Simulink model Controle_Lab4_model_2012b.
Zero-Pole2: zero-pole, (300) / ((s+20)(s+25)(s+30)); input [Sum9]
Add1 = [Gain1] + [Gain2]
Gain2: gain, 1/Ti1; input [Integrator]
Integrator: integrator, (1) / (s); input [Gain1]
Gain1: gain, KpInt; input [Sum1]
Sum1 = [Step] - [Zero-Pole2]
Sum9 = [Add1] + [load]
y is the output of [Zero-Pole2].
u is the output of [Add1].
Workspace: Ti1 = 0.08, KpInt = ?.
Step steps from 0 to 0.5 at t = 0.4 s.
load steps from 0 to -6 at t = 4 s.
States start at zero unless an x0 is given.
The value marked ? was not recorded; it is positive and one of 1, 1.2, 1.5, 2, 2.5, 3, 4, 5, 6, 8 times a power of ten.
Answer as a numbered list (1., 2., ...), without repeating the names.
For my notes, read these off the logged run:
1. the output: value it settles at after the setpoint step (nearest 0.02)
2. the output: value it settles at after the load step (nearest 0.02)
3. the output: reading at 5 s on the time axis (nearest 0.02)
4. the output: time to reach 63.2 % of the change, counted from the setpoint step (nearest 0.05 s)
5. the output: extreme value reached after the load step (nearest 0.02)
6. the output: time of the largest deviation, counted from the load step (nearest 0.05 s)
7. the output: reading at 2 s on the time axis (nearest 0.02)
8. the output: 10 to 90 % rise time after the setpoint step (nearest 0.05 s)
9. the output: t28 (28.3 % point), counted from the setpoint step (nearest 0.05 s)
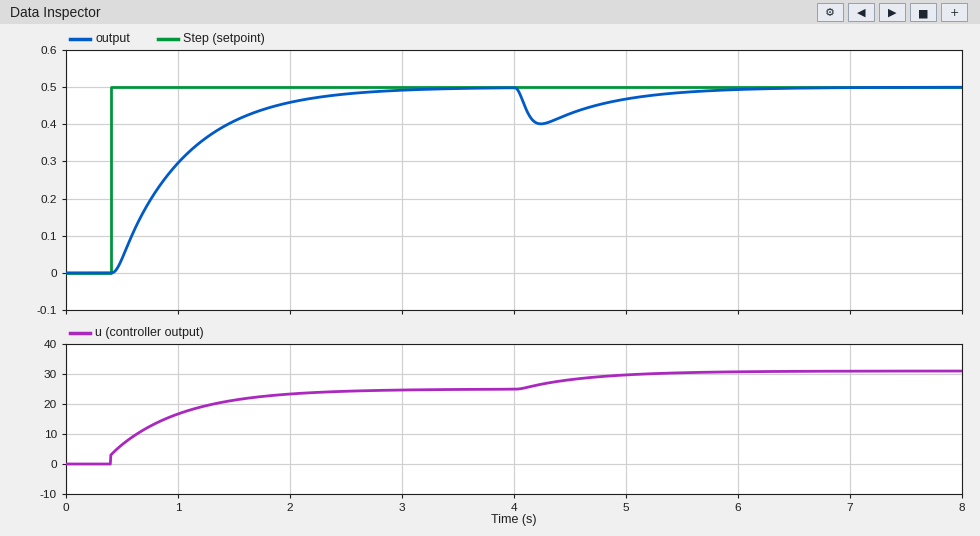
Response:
1. 0.50
2. 0.50
3. 0.46
4. 0.65 s
5. 0.40
6. 0.25 s
7. 0.46
8. 1.35 s
9. 0.25 s
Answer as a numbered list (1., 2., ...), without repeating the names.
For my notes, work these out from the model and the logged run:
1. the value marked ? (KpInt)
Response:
1. 6
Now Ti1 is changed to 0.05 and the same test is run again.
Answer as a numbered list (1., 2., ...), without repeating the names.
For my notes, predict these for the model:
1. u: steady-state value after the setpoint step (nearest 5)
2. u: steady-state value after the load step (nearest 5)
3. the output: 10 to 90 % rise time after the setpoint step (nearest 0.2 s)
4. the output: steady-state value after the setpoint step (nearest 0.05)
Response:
1. 25
2. 30
3. 0.8 s
4. 0.50
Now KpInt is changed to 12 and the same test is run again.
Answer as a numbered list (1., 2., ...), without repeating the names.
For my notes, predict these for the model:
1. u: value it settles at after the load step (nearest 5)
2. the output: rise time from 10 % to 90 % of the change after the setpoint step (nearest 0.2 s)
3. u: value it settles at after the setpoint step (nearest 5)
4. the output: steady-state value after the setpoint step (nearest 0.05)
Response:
1. 30
2. 0.6 s
3. 25
4. 0.50
